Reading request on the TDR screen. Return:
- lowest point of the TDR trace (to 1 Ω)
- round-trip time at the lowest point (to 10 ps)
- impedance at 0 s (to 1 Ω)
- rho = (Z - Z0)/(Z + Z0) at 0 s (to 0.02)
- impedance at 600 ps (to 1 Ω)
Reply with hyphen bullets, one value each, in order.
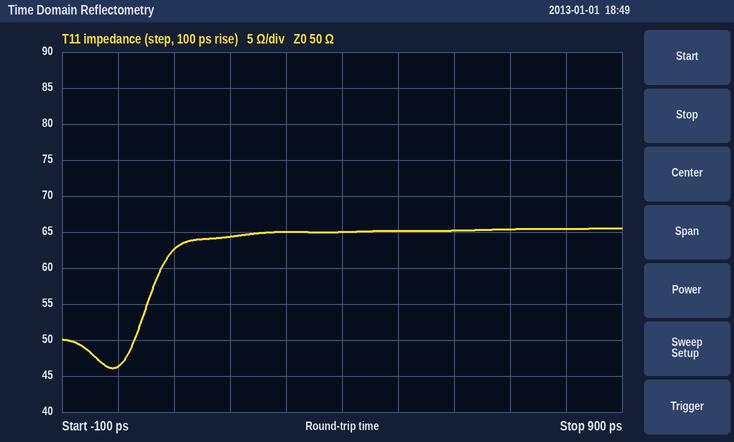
- 46 Ω
- -10 ps
- 46 Ω
- -0.04
- 65 Ω
